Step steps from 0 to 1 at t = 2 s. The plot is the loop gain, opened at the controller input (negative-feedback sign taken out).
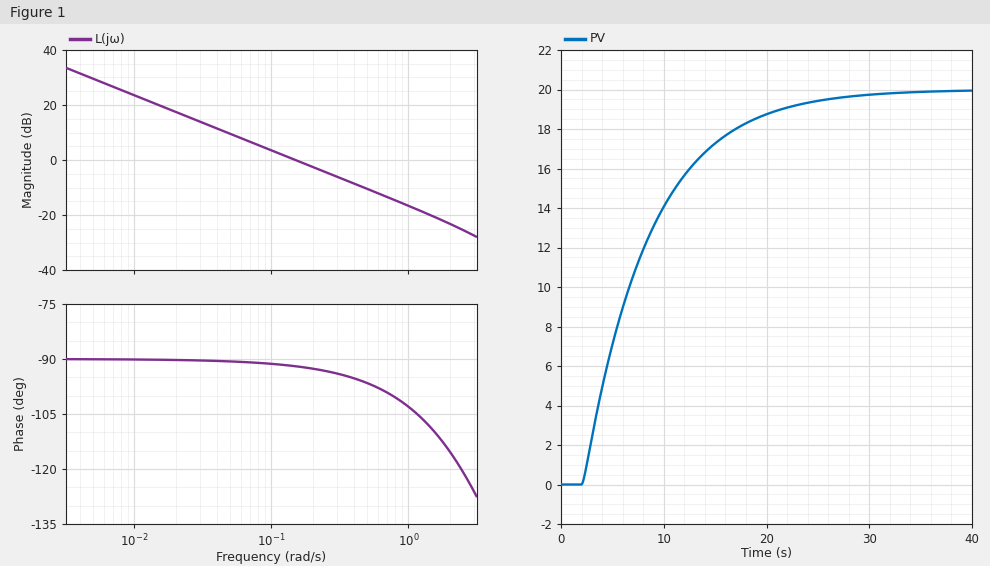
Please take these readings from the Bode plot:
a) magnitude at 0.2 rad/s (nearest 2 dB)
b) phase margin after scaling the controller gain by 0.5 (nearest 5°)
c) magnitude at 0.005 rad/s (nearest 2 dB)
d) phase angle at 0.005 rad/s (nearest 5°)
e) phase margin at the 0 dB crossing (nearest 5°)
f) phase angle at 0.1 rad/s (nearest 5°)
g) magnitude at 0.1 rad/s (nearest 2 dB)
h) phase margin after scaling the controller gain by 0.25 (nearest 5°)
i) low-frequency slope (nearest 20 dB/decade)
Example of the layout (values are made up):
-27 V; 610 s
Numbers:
-2 dB; 90°; 30 dB; -90°; 90°; -90°; 4 dB; 90°; -20 dB/decade
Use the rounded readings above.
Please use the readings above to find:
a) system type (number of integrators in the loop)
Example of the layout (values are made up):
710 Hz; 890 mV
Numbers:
1
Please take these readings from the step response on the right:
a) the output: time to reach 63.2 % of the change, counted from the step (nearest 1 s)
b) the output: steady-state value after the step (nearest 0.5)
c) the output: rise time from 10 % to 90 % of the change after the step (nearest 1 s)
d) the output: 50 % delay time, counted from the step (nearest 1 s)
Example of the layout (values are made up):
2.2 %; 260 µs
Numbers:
7 s; 20.0; 14 s; 5 s
